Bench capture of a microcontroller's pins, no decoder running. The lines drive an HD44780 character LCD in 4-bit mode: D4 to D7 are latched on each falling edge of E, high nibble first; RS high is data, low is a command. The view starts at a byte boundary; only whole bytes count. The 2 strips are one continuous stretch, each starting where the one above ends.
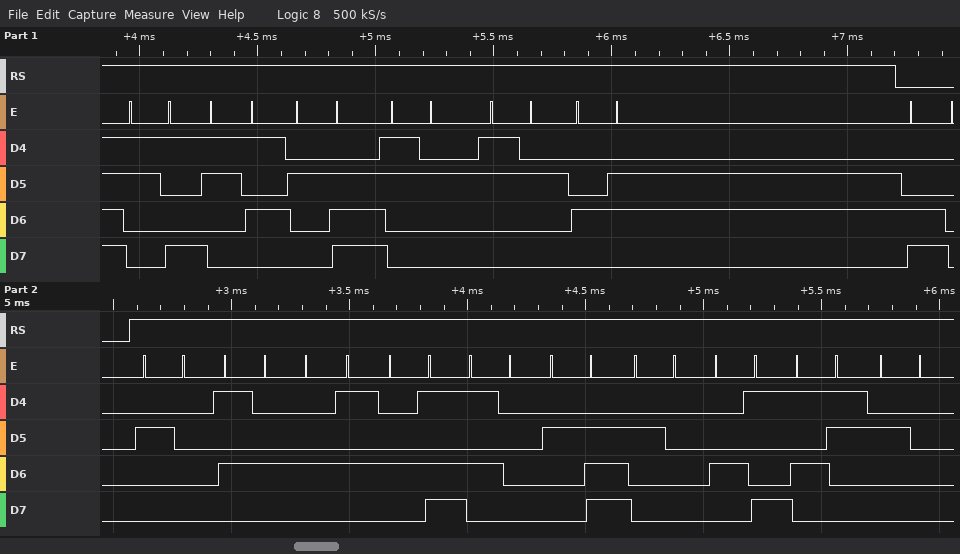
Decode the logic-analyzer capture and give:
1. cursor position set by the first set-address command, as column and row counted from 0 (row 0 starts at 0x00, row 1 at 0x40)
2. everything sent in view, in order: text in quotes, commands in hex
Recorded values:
column 0, row 1
"95.22F" 0xC0 " TEMP. IS "
